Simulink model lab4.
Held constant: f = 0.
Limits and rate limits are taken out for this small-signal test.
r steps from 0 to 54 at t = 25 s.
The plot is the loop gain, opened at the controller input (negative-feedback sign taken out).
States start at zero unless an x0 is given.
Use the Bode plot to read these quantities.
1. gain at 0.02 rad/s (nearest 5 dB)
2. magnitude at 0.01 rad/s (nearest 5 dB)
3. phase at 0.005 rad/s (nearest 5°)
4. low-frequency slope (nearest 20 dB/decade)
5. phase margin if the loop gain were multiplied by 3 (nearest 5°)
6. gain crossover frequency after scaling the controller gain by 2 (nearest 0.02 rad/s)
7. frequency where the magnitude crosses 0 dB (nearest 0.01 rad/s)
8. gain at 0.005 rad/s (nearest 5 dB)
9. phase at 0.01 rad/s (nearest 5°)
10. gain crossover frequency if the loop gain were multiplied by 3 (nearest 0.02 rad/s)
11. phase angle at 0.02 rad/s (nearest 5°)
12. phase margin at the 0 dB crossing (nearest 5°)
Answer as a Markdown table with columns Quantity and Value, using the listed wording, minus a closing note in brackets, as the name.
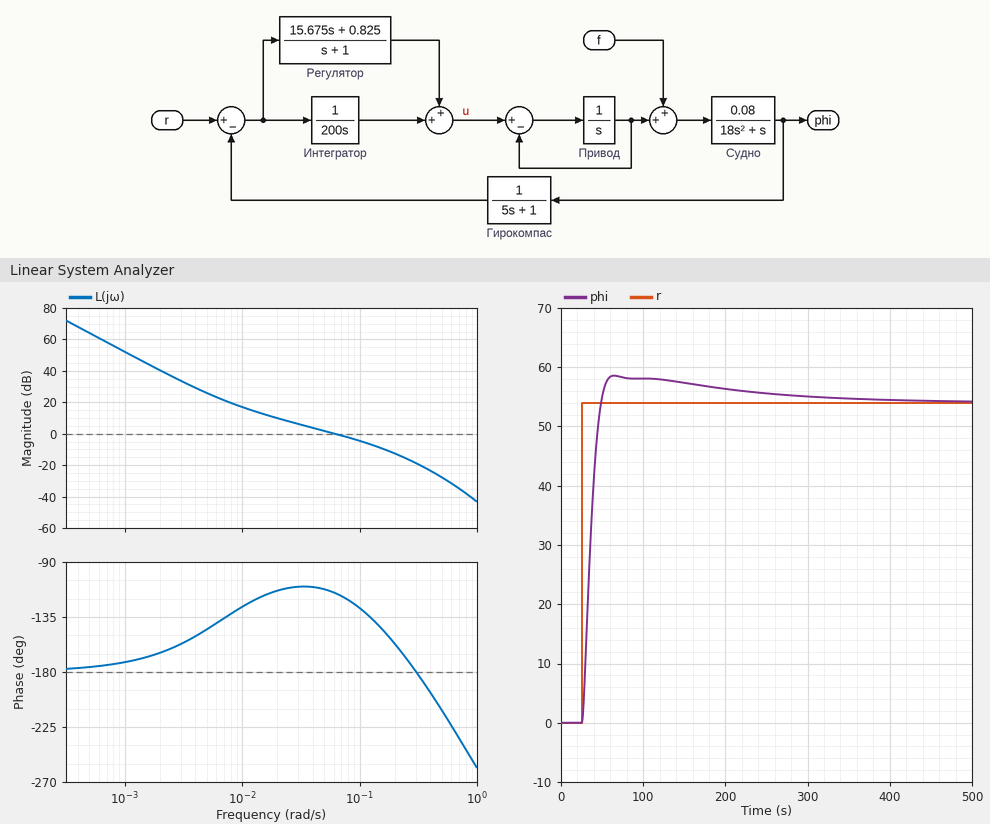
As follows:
| Quantity | Value |
|---|---|
| gain at 0.02 rad/s | 10 dB |
| magnitude at 0.01 rad/s | 15 dB |
| phase at 0.005 rad/s | -145° |
| low-frequency slope | -40 dB/decade |
| phase margin if the loop gain were multiplied by 3 | 35° |
| gain crossover frequency after scaling the controller gain by 2 | 0.12 rad/s |
| frequency where the magnitude crosses 0 dB | 0.06 rad/s |
| gain at 0.005 rad/s | 25 dB |
| phase at 0.01 rad/s | -125° |
| gain crossover frequency if the loop gain were multiplied by 3 | 0.16 rad/s |
| phase angle at 0.02 rad/s | -115° |
| phase margin at the 0 dB crossing | 65° |
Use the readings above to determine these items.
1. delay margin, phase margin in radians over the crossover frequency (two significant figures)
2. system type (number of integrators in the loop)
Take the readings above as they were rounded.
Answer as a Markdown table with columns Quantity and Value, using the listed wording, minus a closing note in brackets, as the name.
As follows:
| Quantity | Value |
|---|---|
| delay margin, phase margin in radians over the crossover frequency | 19 s |
| system type | 2 |
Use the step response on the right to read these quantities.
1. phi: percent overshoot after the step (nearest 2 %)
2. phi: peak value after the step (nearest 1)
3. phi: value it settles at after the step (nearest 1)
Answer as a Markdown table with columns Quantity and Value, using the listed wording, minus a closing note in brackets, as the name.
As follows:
| Quantity | Value |
|---|---|
| phi: percent overshoot after the step | 8 % |
| phi: peak value after the step | 59 |
| phi: value it settles at after the step | 54 |
